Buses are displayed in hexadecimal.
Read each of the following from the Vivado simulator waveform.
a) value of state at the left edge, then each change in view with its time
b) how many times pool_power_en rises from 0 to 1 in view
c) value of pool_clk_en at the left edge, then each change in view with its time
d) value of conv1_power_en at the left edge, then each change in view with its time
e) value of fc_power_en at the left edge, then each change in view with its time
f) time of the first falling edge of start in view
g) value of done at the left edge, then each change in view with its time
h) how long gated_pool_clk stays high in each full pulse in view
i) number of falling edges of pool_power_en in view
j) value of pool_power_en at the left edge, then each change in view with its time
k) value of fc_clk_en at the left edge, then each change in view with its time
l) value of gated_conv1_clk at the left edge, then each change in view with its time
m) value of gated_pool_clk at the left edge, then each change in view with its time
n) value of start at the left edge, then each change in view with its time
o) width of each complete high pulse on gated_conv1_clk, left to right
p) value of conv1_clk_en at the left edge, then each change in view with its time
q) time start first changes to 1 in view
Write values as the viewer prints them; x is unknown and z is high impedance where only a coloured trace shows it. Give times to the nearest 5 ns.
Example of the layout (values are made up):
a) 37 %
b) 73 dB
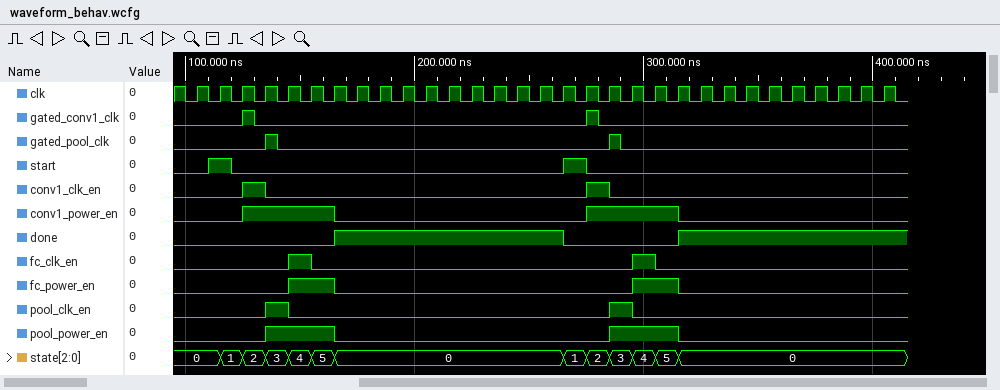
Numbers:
a) 0, 1 at 115 ns, 2 at 125 ns, 3 at 135 ns, 4 at 145 ns, 5 at 155 ns, 0 at 165 ns, 1 at 265 ns, 2 at 275 ns, 3 at 285 ns, 4 at 295 ns, 5 at 305 ns, 0 at 315 ns
b) 2
c) 0, 1 at 135 ns, 0 at 145 ns, 1 at 285 ns, 0 at 295 ns
d) 0, 1 at 125 ns, 0 at 165 ns, 1 at 275 ns, 0 at 315 ns
e) 0, 1 at 145 ns, 0 at 165 ns, 1 at 295 ns, 0 at 315 ns
f) 120 ns
g) 0, 1 at 165 ns, 0 at 265 ns, 1 at 315 ns
h) 5 ns, 5 ns
i) 2
j) 0, 1 at 135 ns, 0 at 165 ns, 1 at 285 ns, 0 at 315 ns
k) 0, 1 at 145 ns, 0 at 155 ns, 1 at 295 ns, 0 at 305 ns
l) 0, 1 at 125 ns, 0 at 130 ns, 1 at 275 ns, 0 at 280 ns
m) 0, 1 at 135 ns, 0 at 140 ns, 1 at 285 ns, 0 at 290 ns
n) 0, 1 at 110 ns, 0 at 120 ns, 1 at 265 ns, 0 at 275 ns
o) 5 ns, 5 ns
p) 0, 1 at 125 ns, 0 at 135 ns, 1 at 275 ns, 0 at 285 ns
q) 110 ns
